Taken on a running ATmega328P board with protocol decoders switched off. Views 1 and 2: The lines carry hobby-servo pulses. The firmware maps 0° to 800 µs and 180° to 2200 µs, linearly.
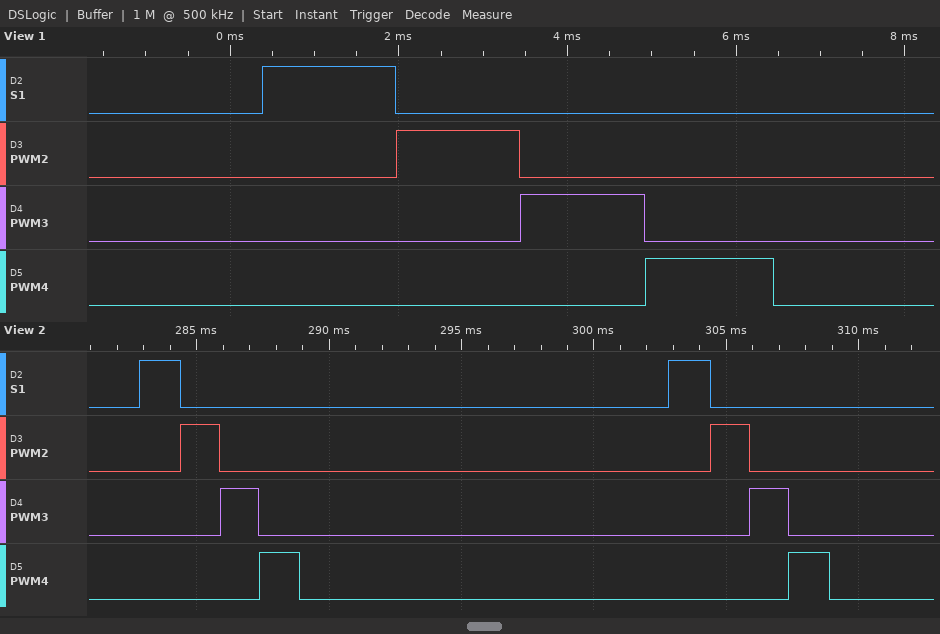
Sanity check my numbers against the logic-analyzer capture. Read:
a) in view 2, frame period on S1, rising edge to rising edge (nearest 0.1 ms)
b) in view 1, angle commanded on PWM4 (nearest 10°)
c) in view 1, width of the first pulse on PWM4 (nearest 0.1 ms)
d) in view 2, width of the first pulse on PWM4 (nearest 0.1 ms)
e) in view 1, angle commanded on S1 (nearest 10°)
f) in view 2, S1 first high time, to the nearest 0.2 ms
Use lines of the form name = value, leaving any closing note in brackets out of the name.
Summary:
in view 2, frame period on S1, rising edge to rising edge = 20.0 ms
in view 1, angle commanded on PWM4 = 90°
in view 1, width of the first pulse on PWM4 = 1.5 ms
in view 2, width of the first pulse on PWM4 = 1.5 ms
in view 1, angle commanded on S1 = 100°
in view 2, S1 first high time, to the nearest 0.2 ms = 1.6 ms
